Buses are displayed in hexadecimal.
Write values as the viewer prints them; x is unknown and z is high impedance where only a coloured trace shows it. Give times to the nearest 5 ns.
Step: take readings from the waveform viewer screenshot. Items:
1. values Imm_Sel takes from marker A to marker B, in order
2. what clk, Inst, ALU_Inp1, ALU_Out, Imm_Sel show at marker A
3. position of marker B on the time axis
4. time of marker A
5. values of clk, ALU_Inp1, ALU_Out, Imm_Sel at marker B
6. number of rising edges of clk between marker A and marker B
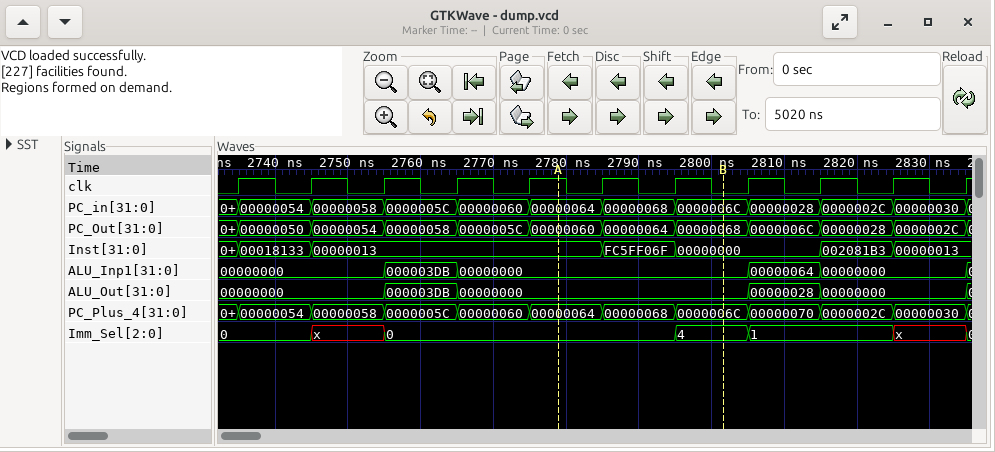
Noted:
0, 4
clk=1, Inst=00000013, ALU_Inp1=00000000, ALU_Out=00000000, Imm_Sel=0
2800 ns
2780 ns
clk=0, ALU_Inp1=00000000, ALU_Out=00000000, Imm_Sel=4
2
